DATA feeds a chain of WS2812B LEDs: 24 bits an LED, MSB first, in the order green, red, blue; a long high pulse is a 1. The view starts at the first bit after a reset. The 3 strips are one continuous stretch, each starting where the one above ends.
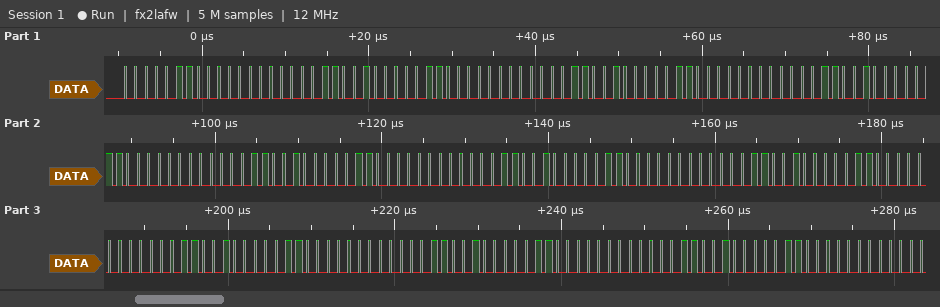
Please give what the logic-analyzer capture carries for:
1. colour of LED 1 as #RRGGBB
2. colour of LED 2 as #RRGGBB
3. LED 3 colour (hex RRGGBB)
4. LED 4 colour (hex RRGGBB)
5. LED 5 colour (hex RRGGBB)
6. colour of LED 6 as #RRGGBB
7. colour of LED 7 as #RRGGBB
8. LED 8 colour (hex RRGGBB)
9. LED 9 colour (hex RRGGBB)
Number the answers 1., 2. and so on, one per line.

1. #000619
2. #000619
3. #000619
4. #000619
5. #000619
6. #000619
7. #000619
8. #000619
9. #000619
